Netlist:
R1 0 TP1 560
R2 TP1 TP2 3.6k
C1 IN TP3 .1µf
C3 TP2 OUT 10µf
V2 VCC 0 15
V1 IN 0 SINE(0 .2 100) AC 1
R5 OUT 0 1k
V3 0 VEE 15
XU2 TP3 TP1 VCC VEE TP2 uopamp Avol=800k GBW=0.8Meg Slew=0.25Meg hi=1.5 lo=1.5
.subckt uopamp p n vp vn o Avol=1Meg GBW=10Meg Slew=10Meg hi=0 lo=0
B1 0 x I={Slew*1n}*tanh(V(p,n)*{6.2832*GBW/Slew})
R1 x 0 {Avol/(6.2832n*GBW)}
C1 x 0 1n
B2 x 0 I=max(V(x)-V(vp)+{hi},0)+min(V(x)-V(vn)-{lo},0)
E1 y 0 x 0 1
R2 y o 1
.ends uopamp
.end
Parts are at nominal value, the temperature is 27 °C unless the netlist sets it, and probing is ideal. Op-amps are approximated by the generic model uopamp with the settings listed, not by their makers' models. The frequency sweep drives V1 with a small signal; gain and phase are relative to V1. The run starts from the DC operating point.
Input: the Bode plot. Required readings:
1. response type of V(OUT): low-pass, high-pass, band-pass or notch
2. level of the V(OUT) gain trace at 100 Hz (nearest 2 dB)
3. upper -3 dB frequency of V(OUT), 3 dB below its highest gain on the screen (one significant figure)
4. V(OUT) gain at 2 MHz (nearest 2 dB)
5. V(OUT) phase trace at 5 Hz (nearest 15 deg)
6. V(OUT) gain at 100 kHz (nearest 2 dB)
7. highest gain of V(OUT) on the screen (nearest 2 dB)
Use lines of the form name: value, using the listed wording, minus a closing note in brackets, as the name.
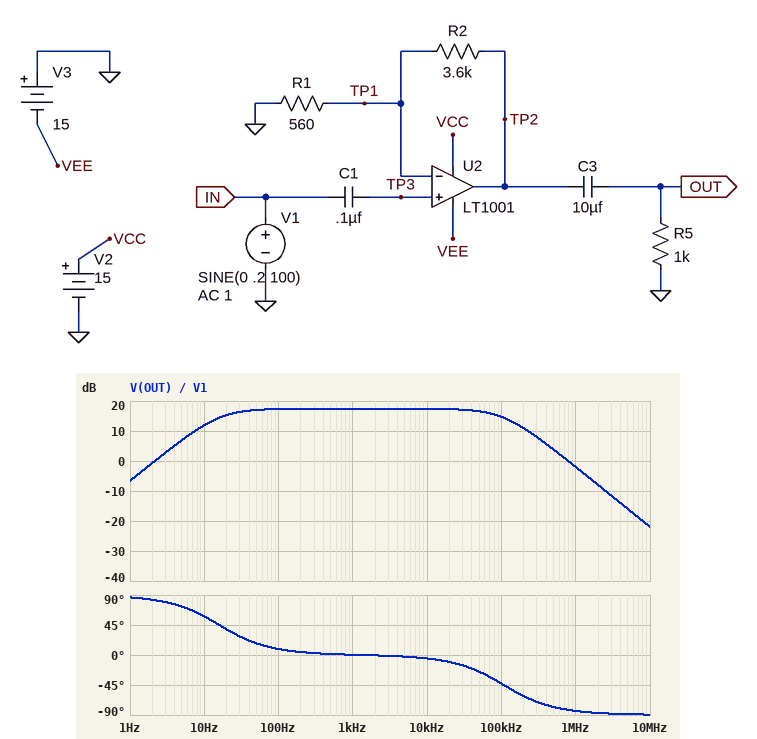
response type of V(OUT): low-pass, high-pass, band-pass or notch: band-pass
level of the V(OUT) gain trace at 100 Hz: 18 dB
upper -3 dB frequency of V(OUT), 3 dB below its highest gain on the screen: 100 kHz
V(OUT) gain at 2 MHz: -8 dB
V(OUT) phase trace at 5 Hz: 75 deg
V(OUT) gain at 100 kHz: 14 dB
highest gain of V(OUT) on the screen: 18 dB
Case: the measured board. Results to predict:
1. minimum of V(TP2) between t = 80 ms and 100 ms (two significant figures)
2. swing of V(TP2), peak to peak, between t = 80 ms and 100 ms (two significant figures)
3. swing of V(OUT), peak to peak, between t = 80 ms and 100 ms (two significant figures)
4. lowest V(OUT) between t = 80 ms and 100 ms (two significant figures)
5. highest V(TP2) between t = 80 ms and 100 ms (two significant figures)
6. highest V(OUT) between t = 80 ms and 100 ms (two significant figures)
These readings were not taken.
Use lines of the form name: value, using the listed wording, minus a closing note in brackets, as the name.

minimum of V(TP2) between t = 80 ms and 100 ms: -1.5 V
swing of V(TP2), peak to peak, between t = 80 ms and 100 ms: 3.0 V
swing of V(OUT), peak to peak, between t = 80 ms and 100 ms: 2.9 V
lowest V(OUT) between t = 80 ms and 100 ms: -1.5 V
highest V(TP2) between t = 80 ms and 100 ms: 1.5 V
highest V(OUT) between t = 80 ms and 100 ms: 1.5 V
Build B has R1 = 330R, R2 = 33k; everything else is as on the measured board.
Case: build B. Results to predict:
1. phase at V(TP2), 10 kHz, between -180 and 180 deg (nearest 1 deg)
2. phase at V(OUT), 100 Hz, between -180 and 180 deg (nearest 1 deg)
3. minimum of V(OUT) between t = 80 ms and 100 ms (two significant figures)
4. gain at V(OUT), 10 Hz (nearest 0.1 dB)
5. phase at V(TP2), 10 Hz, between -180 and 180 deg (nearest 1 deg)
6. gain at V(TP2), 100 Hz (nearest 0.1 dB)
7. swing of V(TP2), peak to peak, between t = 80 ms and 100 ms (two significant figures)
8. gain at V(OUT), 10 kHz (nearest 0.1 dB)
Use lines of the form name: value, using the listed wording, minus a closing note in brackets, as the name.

phase at V(TP2), 10 kHz, between -180 and 180 deg: -52 deg
phase at V(OUT), 100 Hz, between -180 and 180 deg: 8 deg
minimum of V(OUT) between t = 80 ms and 100 ms: -15 V
gain at V(OUT), 10 Hz: 34.6 dB
phase at V(TP2), 10 Hz, between -180 and 180 deg: 0 deg
gain at V(TP2), 100 Hz: 40.1 dB
swing of V(TP2), peak to peak, between t = 80 ms and 100 ms: 27 V
gain at V(OUT), 10 kHz: 35.9 dB
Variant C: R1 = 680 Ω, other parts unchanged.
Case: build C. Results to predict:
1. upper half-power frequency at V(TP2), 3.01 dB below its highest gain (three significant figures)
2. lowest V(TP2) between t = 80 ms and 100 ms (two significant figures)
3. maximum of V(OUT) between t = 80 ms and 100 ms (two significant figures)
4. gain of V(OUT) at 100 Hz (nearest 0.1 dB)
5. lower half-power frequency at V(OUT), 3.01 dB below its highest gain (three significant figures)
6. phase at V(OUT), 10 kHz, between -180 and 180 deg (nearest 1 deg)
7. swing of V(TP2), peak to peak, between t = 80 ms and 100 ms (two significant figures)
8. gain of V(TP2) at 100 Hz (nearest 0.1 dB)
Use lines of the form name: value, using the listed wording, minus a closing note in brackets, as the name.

upper half-power frequency at V(TP2), 3.01 dB below its highest gain: 127 kHz
lowest V(TP2) between t = 80 ms and 100 ms: -1.3 V
maximum of V(OUT) between t = 80 ms and 100 ms: 1.2 V
gain of V(OUT) at 100 Hz: 15.9 dB
lower half-power frequency at V(OUT), 3.01 dB below its highest gain: 15.9 Hz
phase at V(OUT), 10 kHz, between -180 and 180 deg: -4 deg
swing of V(TP2), peak to peak, between t = 80 ms and 100 ms: 2.5 V
gain of V(TP2) at 100 Hz: 16.0 dB
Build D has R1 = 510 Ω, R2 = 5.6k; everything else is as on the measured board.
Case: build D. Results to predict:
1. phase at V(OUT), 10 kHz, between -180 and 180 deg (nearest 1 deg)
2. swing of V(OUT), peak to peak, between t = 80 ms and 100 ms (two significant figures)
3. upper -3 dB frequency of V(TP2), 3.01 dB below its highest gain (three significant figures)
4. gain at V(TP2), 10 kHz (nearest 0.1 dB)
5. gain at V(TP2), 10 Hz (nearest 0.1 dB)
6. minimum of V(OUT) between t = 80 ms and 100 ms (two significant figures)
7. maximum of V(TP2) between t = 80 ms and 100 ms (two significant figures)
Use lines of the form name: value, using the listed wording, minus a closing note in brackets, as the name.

phase at V(OUT), 10 kHz, between -180 and 180 deg: -8 deg
swing of V(OUT), peak to peak, between t = 80 ms and 100 ms: 4.7 V
upper -3 dB frequency of V(TP2), 3.01 dB below its highest gain: 66.7 kHz
gain at V(TP2), 10 kHz: 21.5 dB
gain at V(TP2), 10 Hz: 21.6 dB
minimum of V(OUT) between t = 80 ms and 100 ms: -2.4 V
maximum of V(TP2) between t = 80 ms and 100 ms: 2.4 V
